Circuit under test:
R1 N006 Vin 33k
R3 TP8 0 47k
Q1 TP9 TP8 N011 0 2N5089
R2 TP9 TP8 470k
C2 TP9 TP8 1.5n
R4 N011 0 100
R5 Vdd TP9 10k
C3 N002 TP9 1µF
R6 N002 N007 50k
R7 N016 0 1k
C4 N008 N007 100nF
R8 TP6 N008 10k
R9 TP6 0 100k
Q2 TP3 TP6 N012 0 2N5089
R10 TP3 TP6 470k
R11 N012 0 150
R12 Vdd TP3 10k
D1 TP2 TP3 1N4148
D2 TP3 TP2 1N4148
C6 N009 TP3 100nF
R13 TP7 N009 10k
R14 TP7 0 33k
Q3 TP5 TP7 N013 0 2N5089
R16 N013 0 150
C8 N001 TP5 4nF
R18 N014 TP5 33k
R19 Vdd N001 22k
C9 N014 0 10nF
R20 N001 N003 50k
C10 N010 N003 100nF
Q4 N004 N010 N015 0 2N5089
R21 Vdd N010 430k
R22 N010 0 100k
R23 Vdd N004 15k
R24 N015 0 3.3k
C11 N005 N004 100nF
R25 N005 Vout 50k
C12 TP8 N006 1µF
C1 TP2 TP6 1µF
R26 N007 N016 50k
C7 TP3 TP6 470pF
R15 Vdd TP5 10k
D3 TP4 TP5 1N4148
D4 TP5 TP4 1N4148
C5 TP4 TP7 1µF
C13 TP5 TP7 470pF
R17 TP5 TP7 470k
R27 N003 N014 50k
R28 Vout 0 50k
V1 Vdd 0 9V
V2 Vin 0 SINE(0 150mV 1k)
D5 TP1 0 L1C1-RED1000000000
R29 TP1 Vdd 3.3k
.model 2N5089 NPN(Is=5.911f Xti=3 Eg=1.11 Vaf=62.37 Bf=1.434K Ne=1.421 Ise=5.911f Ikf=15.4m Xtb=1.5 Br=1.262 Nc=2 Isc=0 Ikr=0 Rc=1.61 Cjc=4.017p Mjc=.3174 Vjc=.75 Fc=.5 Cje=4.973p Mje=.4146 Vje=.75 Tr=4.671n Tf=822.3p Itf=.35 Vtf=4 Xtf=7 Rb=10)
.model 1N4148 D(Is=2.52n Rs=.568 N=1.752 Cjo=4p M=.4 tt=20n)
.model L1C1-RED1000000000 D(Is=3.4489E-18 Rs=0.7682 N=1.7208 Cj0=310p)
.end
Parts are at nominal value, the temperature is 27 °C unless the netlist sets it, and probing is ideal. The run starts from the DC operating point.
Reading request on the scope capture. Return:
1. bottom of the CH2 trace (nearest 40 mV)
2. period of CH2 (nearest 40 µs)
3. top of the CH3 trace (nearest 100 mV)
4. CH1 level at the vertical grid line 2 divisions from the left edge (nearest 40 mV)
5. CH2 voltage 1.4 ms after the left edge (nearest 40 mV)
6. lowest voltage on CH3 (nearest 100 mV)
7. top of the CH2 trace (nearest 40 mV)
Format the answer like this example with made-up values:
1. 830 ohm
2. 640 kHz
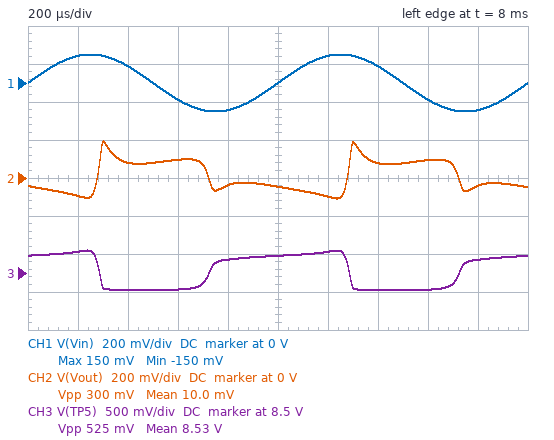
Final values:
1. -120 mV
2. 1.00 ms
3. 8.8 V
4. 80 mV
5. 80 mV
6. 8.3 V
7. 200 mV
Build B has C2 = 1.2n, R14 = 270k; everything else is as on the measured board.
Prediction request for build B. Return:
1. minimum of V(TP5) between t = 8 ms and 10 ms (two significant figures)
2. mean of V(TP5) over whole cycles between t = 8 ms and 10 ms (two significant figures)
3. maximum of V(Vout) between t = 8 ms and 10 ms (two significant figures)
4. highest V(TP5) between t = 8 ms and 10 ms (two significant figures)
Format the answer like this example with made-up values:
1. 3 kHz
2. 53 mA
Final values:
1. 2.1 V
2. 2.5 V
3. 270 mV
4. 2.9 V
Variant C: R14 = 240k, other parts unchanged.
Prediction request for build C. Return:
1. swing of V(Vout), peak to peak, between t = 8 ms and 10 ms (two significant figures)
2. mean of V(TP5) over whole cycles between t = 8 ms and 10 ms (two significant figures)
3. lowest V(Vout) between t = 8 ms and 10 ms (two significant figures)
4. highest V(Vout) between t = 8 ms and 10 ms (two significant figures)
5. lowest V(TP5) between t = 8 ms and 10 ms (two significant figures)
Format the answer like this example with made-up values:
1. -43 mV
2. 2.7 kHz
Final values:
1. 530 mV
2. 2.6 V
3. -270 mV
4. 260 mV
5. 2.2 V
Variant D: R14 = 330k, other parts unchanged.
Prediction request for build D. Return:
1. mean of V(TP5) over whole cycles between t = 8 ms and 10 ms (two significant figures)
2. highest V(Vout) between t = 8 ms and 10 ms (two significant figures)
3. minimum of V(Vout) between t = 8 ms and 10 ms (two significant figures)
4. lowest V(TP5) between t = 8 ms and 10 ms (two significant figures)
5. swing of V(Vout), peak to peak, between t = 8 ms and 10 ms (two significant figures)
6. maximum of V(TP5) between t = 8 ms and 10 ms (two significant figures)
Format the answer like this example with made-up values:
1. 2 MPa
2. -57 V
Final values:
1. 2.3 V
2. 260 mV
3. -270 mV
4. 1.9 V
5. 530 mV
6. 2.7 V
